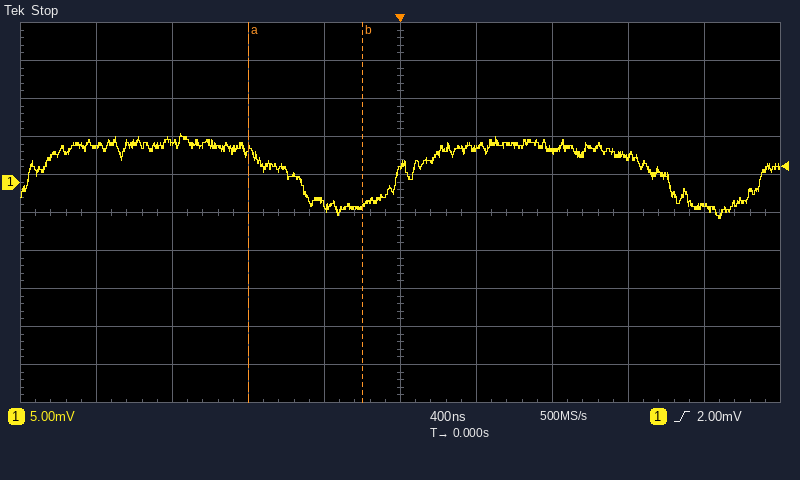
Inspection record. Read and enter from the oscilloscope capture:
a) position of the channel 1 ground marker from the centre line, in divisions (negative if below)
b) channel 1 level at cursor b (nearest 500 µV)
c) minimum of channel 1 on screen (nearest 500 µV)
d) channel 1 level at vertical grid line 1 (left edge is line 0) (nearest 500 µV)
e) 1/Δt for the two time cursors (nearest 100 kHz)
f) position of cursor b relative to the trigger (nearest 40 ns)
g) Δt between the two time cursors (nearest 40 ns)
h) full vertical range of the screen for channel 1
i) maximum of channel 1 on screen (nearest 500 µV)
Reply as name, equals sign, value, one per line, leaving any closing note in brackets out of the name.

position of the channel 1 ground marker from the centre line, in divisions = +0.8 div
channel 1 level at cursor b = -3.0 mV
minimum of channel 1 on screen = -5.0 mV
channel 1 level at vertical grid line 1 (left edge is line 0) = 5.0 mV
1/Δt for the two time cursors = 1.7 MHz
position of cursor b relative to the trigger = -200 ns
Δt between the two time cursors = 600 ns
full vertical range of the screen for channel 1 = 50 mV
maximum of channel 1 on screen = 6.5 mV
